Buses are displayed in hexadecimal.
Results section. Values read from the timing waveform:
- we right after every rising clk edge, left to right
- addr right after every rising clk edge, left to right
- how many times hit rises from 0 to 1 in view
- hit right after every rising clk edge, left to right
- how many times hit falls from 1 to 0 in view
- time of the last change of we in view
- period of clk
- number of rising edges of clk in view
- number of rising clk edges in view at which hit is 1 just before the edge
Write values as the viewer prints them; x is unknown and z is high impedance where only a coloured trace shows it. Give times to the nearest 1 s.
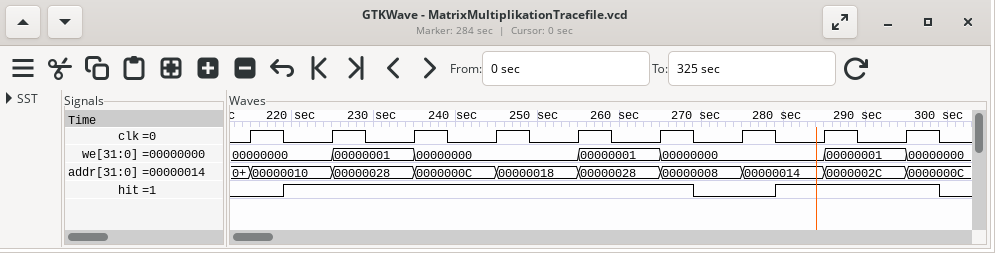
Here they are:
00000000, 00000001, 00000000, 00000000, 00000001, 00000000, 00000000, 00000001, 00000000
00000010, 00000028, 0000000C, 00000018, 00000028, 00000008, 00000014, 0000002C, 0000000C
2
0 1 1 1 1 1 0 1 1
2
295 s
10 s
9
7
